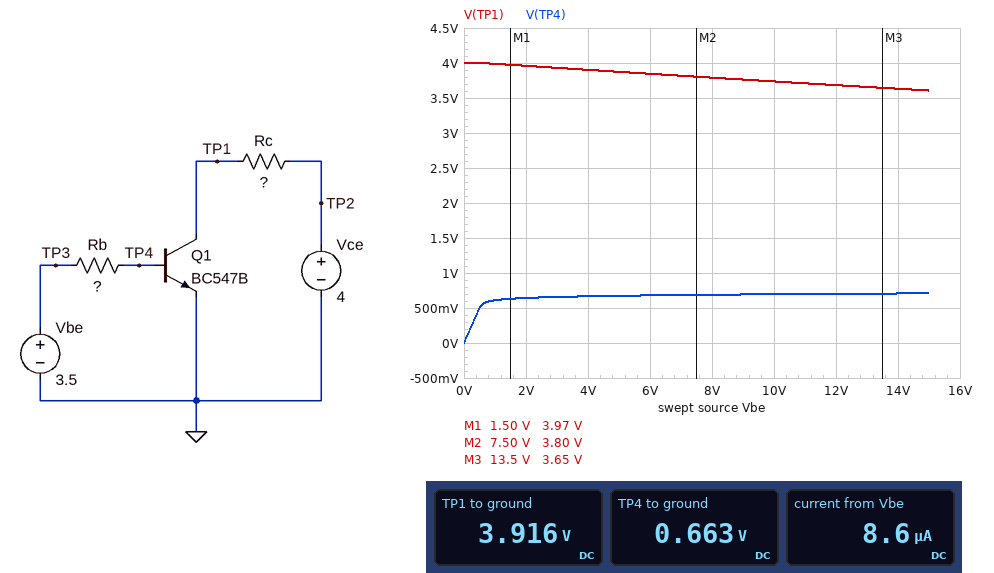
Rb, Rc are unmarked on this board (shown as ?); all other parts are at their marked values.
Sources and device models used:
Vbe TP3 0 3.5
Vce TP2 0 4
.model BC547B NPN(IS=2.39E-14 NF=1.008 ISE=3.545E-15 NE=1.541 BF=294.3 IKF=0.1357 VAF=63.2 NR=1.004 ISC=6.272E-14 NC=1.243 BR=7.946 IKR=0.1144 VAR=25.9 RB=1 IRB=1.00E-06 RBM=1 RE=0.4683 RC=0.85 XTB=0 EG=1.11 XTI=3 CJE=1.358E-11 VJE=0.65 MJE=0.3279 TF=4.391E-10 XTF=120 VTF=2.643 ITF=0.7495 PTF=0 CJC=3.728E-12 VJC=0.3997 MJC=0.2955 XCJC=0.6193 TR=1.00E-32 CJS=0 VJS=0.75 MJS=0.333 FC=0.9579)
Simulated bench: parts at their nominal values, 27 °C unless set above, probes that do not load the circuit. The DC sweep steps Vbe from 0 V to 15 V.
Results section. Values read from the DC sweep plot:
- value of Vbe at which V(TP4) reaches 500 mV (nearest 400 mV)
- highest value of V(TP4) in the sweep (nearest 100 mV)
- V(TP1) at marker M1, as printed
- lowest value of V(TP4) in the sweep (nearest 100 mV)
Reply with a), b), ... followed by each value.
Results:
a) 400 mV
b) 700 mV
c) 3.97 V
d) 0 V
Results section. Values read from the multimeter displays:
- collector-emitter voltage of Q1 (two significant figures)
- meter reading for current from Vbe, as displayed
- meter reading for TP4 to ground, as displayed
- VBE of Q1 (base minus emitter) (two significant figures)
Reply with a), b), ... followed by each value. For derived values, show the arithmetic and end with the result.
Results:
a) 3.916 V = 3.9 V
b) 8.6 µA
c) 0.663 V
d) 663 mV = 660 mV
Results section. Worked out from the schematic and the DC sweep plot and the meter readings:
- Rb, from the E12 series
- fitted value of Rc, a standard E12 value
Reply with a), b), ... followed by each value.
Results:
a) 330 kΩ
b) 33 Ω
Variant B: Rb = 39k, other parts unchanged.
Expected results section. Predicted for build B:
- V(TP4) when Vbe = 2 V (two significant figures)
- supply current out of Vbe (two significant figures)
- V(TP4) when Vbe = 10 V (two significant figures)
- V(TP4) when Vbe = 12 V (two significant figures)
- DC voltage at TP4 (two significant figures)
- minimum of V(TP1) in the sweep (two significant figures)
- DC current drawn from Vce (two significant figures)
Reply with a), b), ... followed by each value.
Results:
a) 700 mV
b) 71 µA
c) 770 mV
d) 780 mV
e) 730 mV
f) 1.7 V
g) 19 mA
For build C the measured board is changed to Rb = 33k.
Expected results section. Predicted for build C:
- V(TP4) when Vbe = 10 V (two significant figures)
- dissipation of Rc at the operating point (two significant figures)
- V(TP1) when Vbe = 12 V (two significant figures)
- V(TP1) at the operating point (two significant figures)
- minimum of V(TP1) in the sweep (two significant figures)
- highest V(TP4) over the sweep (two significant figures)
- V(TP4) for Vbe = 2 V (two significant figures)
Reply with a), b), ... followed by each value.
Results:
a) 780 mV
b) 15 mW
c) 1.8 V
d) 3.3 V
e) 1.4 V
f) 800 mV
g) 710 mV
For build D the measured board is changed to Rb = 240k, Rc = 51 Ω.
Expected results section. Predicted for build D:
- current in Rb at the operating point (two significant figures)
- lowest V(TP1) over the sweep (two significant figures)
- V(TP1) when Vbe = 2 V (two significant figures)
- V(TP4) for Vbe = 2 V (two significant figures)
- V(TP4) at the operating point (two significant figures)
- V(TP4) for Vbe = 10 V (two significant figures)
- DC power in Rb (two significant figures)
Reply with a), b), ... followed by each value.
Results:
a) 12 µA
b) 3.2 V
c) 3.9 V
d) 650 mV
e) 670 mV
f) 710 mV
g) 33 µW
